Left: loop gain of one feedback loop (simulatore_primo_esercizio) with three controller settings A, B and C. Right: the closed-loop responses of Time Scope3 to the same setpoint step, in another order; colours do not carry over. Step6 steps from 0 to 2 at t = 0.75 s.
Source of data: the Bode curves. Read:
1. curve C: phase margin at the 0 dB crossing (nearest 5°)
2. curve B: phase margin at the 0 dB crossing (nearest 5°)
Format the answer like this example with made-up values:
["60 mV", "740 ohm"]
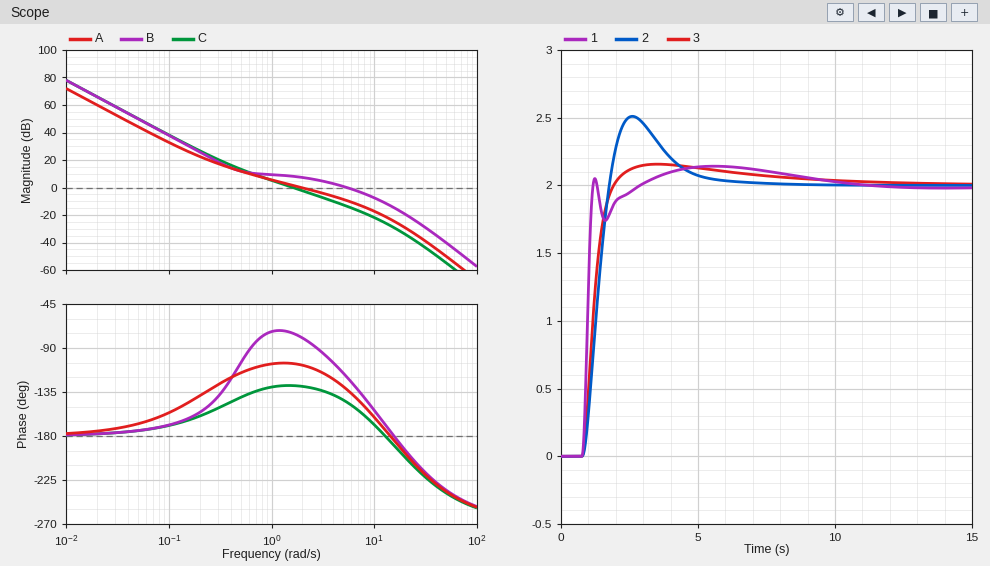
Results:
["50°", "60°"]
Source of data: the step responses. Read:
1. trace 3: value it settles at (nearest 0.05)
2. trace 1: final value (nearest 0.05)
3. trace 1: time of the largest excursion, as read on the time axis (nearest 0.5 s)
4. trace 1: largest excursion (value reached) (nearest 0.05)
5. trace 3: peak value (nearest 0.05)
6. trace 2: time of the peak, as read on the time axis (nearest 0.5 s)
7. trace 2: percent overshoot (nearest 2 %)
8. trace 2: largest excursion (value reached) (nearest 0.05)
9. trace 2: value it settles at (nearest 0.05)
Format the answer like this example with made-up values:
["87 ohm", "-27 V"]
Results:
["2.00", "2.00", "5.5 s", "2.15", "2.15", "2.5 s", "26 %", "2.50", "2.00"]
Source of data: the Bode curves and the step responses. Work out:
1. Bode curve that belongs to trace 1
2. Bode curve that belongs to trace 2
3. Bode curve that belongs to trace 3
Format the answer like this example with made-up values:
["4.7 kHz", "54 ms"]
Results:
["B", "C", "A"]
